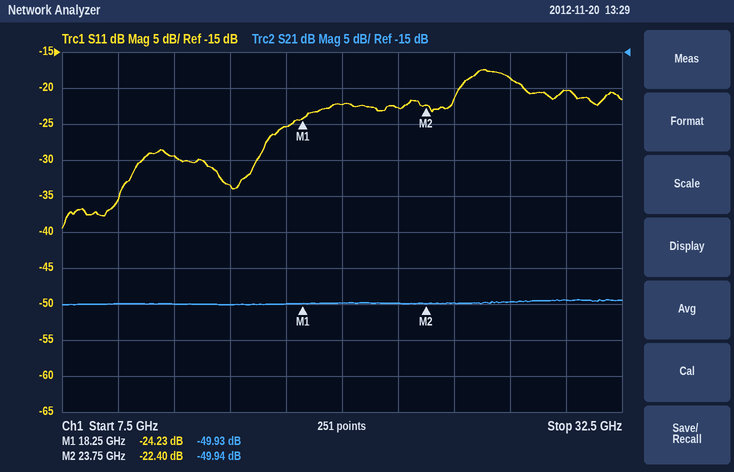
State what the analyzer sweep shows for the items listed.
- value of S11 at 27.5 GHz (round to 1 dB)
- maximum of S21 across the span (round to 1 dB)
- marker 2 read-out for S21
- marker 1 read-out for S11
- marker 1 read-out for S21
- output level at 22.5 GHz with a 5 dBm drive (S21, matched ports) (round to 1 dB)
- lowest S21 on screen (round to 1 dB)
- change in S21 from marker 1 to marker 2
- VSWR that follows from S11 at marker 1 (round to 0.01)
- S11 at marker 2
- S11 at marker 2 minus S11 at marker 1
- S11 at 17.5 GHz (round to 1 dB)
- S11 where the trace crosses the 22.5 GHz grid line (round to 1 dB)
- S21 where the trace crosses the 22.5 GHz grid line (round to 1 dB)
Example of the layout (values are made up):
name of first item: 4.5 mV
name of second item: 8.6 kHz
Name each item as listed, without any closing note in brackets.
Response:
value of S11 at 27.5 GHz: -19 dB
maximum of S21 across the span: -49 dB
marker 2 read-out for S21: -49.94 dB
marker 1 read-out for S11: -24.23 dB
marker 1 read-out for S21: -49.93 dB
output level at 22.5 GHz with a 5 dBm drive (S21, matched ports): -45 dBm
lowest S21 on screen: -50 dB
change in S21 from marker 1 to marker 2: -0.01 dB
VSWR that follows from S11 at marker 1: 1.13
S11 at marker 2: -22.40 dB
S11 at marker 2 minus S11 at marker 1: 1.83 dB
S11 at 17.5 GHz: -25 dB
S11 where the trace crosses the 22.5 GHz grid line: -23 dB
S21 where the trace crosses the 22.5 GHz grid line: -50 dB
